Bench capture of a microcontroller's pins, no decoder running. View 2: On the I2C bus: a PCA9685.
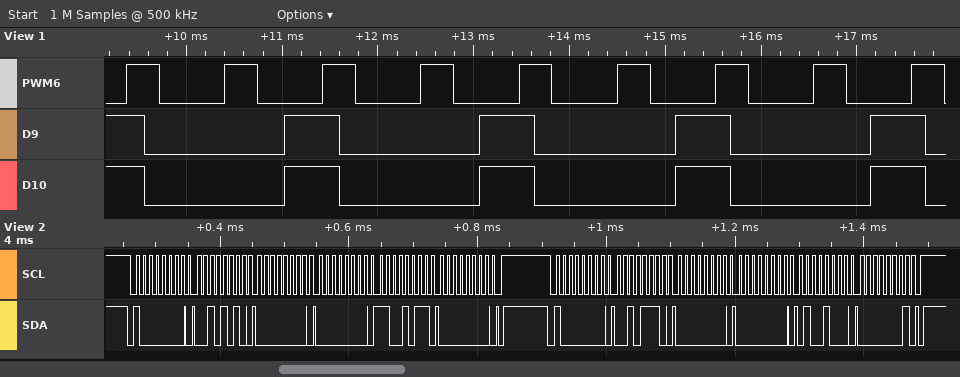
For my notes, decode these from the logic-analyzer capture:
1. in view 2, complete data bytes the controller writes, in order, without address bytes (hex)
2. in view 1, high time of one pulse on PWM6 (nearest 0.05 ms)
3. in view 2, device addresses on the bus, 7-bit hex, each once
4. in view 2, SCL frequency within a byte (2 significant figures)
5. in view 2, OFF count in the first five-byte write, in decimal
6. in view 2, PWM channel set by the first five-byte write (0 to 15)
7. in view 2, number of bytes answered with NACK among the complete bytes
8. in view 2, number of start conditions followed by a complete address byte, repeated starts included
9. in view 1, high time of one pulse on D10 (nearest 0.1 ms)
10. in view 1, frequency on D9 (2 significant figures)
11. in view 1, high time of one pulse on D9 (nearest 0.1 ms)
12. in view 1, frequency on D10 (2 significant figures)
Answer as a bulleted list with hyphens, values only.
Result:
- 2A 00 00 CB 00 2E 00 00 48 01
- 0.35 ms
- 0x40
- 100 kHz
- 203
- 9
- 0
- 2
- 0.6 ms
- 490 Hz
- 0.6 ms
- 490 Hz
